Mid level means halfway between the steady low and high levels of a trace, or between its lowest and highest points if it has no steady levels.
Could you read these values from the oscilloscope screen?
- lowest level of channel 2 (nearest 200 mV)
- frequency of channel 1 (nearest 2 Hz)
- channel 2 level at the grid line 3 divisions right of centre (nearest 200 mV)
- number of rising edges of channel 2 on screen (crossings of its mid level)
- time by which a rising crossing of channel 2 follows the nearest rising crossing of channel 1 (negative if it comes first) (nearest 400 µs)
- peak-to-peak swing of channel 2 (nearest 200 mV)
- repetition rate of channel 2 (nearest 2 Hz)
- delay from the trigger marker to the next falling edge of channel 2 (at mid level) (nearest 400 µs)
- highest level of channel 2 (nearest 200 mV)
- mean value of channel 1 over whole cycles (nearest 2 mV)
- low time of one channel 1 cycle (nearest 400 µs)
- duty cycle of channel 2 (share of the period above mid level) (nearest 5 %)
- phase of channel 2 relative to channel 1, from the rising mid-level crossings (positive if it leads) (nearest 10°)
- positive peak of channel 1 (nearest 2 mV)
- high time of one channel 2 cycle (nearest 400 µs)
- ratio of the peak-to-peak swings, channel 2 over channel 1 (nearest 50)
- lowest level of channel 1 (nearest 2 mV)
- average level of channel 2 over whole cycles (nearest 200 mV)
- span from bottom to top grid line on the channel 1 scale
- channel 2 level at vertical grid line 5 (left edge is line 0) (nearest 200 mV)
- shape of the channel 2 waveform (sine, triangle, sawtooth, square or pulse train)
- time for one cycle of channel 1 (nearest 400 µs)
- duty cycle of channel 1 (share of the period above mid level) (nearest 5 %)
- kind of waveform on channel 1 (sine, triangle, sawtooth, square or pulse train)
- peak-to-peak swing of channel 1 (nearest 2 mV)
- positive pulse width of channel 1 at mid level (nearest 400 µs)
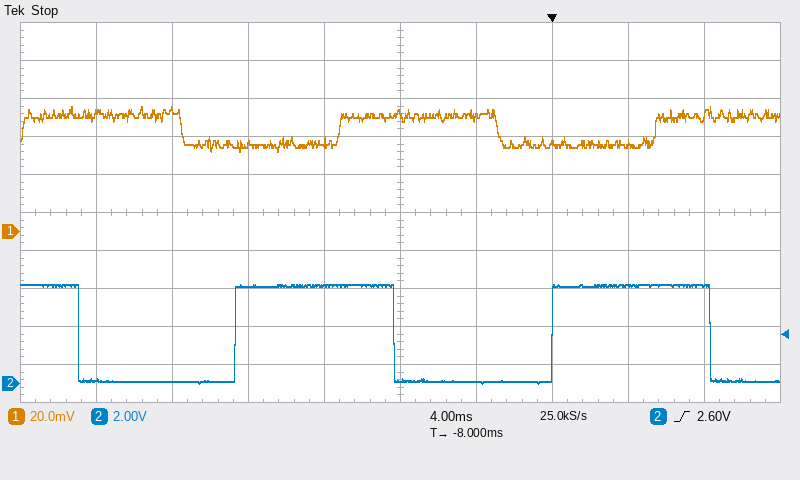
0.0 V
60 Hz
5.2 V
2
-5.6 ms
5.2 V
60 Hz
8.4 ms
5.2 V
54 mV
8.4 ms
50 %
+120°
66 mV
8.4 ms
200
42 mV
2.6 V
200 mV
200 mV
square
16.8 ms
50 %
square
24 mV
8.4 ms
